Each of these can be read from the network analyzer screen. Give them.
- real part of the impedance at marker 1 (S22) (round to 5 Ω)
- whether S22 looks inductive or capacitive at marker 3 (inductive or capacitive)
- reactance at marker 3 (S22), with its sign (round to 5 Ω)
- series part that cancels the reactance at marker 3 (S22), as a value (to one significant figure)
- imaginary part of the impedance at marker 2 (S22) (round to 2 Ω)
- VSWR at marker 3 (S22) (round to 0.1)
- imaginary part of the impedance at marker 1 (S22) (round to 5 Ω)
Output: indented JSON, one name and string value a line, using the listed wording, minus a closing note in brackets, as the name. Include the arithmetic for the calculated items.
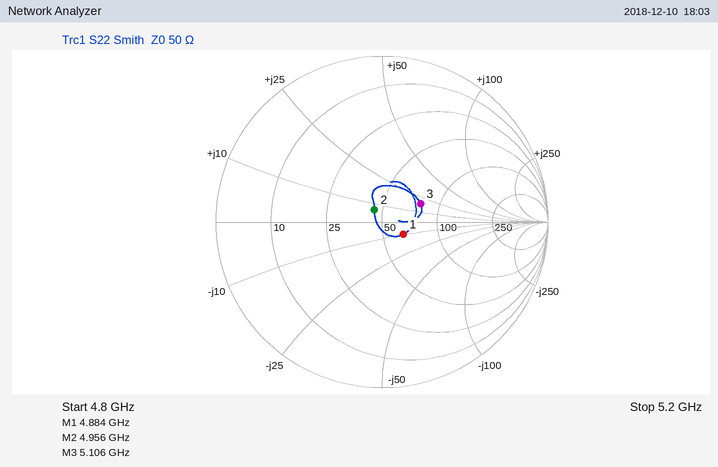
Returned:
{
  "real part of the impedance at marker 1 (S22)": "65 Ω",
  "whether S22 looks inductive or capacitive at marker 3": "inductive",
  "reactance at marker 3 (S22), with its sign": "+20 Ω",
  "series part that cancels the reactance at marker 3 (S22), as a value": "C = 1/(2π × 5.106 GHz × 20 Ω) ≈ 2 pF",
  "imaginary part of the impedance at marker 2 (S22)": "+6 Ω",
  "VSWR at marker 3 (S22)": "1.7",
  "imaginary part of the impedance at marker 1 (S22)": "-10 Ω"
}
